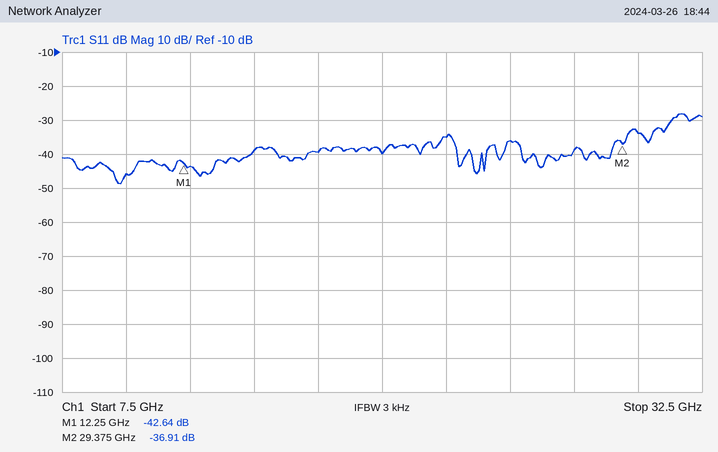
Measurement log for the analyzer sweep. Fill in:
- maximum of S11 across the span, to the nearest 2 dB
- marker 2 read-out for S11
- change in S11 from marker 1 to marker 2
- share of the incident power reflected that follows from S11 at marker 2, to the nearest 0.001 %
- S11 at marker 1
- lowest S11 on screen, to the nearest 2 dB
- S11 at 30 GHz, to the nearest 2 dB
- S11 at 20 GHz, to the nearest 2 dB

-28 dB
-36.91 dB
5.73 dB
0.020 %
-42.64 dB
-48 dB
-34 dB
-40 dB
